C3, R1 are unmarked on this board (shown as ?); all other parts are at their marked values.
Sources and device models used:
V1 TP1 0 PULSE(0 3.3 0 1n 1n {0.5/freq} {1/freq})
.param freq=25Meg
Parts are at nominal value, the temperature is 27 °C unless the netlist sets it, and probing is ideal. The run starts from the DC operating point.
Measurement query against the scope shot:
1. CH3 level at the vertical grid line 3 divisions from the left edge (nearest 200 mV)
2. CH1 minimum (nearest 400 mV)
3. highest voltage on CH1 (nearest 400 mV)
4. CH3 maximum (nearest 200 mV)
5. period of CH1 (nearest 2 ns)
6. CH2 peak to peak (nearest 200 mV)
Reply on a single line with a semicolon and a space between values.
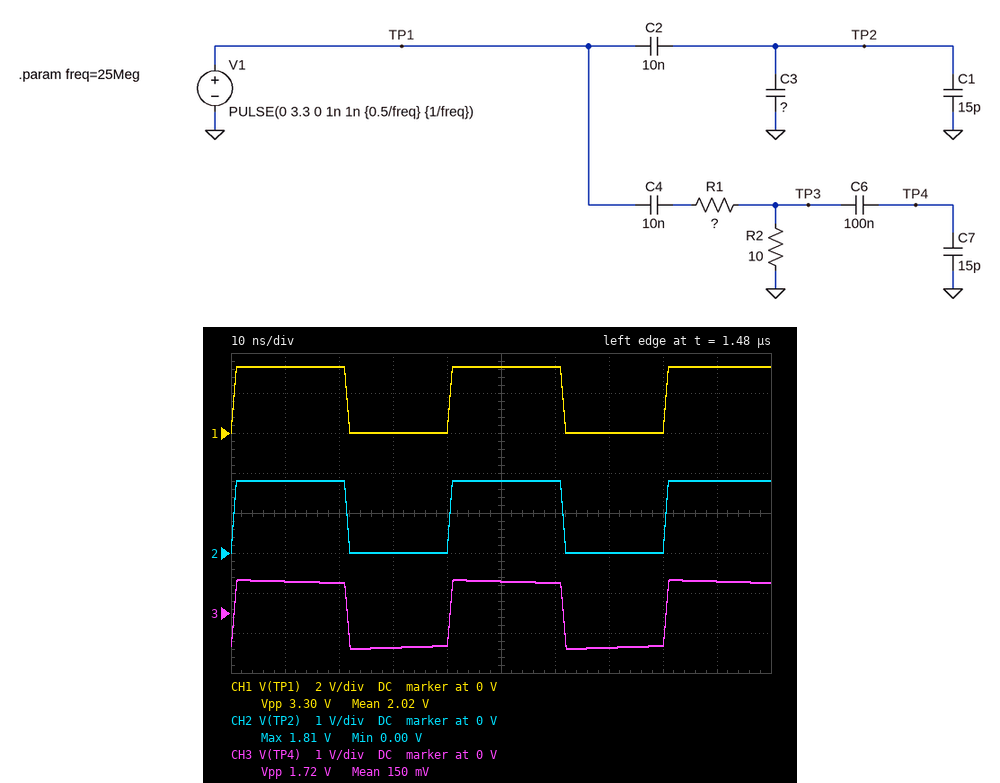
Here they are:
-800 mV; 0 V; 3.2 V; 800 mV; 40 ns; 1.8 V
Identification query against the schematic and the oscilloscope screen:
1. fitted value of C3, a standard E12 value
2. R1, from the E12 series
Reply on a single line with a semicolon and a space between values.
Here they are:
8.2 nF; 10 Ω
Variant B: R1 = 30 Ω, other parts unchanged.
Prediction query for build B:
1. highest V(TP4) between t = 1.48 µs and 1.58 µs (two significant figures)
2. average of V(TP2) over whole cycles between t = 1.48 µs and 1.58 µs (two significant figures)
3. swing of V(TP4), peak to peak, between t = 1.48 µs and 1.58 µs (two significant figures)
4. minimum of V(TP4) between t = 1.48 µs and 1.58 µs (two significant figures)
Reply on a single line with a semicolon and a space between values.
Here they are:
410 mV; 950 mV; 840 mV; -430 mV
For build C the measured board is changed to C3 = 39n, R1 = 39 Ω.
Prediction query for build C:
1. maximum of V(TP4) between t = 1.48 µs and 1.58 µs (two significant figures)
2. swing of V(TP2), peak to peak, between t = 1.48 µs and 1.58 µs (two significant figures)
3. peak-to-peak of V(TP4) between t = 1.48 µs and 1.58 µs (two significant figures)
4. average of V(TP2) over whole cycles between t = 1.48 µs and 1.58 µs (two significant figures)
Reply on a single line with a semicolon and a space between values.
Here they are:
340 mV; 670 mV; 690 mV; 350 mV
